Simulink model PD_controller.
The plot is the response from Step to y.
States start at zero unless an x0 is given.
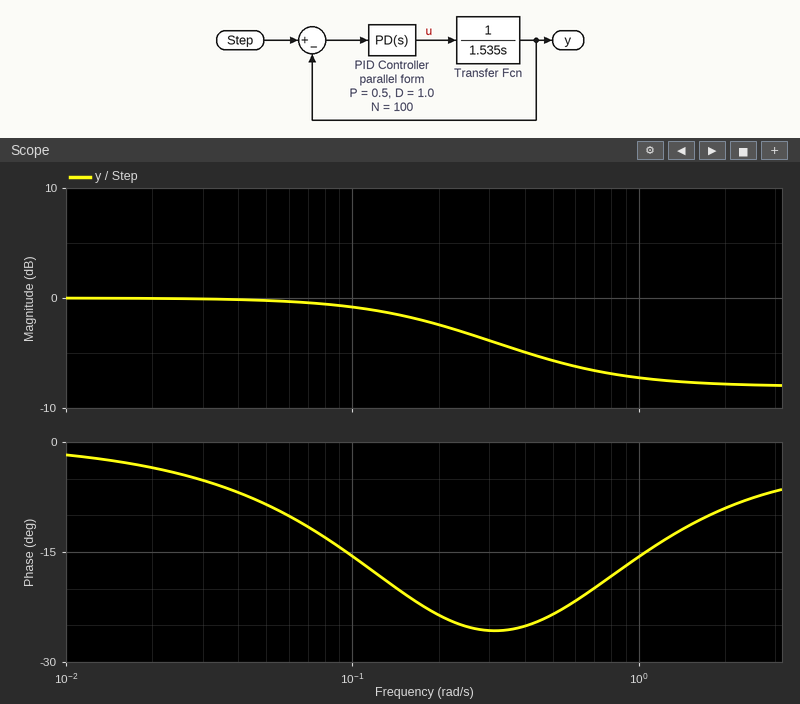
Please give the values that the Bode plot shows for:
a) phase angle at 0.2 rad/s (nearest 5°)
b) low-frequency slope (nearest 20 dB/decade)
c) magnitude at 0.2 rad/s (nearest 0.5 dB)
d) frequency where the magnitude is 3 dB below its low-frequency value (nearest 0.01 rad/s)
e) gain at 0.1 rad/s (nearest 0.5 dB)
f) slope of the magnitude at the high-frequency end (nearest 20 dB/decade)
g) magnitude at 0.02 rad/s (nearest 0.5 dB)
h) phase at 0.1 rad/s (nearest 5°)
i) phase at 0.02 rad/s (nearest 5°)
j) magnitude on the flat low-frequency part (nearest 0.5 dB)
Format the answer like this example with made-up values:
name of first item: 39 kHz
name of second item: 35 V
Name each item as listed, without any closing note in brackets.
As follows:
phase angle at 0.2 rad/s: -25°
low-frequency slope: 0 dB/decade
magnitude at 0.2 rad/s: -2.5 dB
frequency where the magnitude is 3 dB below its low-frequency value: 0.24 rad/s
gain at 0.1 rad/s: -1.0 dB
slope of the magnitude at the high-frequency end: 0 dB/decade
magnitude at 0.02 rad/s: 0.0 dB
phase at 0.1 rad/s: -15°
phase at 0.02 rad/s: -5°
magnitude on the flat low-frequency part: 0.0 dB
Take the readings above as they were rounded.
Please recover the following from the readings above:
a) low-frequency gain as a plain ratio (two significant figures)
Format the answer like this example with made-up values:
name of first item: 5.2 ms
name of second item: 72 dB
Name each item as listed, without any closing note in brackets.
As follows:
low-frequency gain as a plain ratio: 1.0
